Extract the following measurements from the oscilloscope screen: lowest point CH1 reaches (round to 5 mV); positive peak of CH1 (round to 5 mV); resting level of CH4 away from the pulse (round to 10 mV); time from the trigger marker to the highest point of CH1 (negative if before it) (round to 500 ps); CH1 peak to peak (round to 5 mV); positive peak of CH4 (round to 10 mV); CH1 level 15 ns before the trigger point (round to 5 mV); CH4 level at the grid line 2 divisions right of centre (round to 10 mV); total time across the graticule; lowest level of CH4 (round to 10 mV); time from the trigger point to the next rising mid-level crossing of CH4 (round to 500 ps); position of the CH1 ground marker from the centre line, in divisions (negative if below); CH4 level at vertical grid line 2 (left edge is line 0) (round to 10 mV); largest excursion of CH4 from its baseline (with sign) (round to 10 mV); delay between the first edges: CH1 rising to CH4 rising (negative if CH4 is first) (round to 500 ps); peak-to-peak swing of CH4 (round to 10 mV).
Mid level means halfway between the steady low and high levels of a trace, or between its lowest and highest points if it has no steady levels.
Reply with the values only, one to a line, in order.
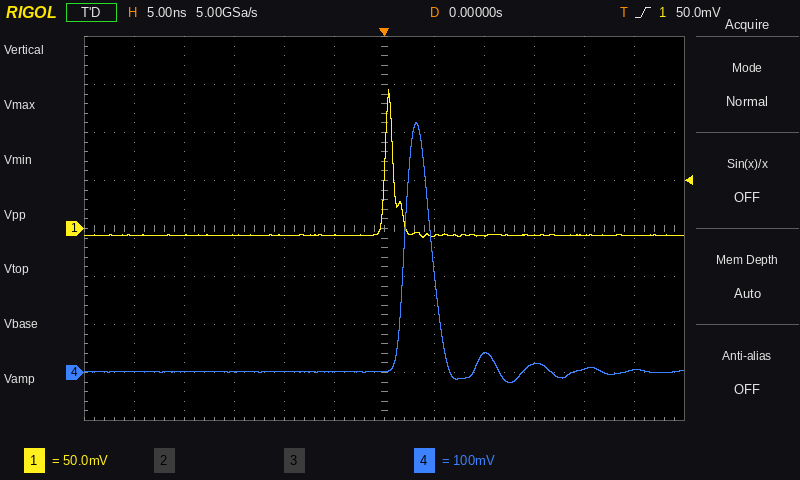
-10 mV
145 mV
0 mV
+500 ps
155 mV
520 mV
-5 mV
40 mV
60 ns
-20 mV
2.0 ns
0.0 div
0 mV
+520 mV
+2.0 ns
540 mV
